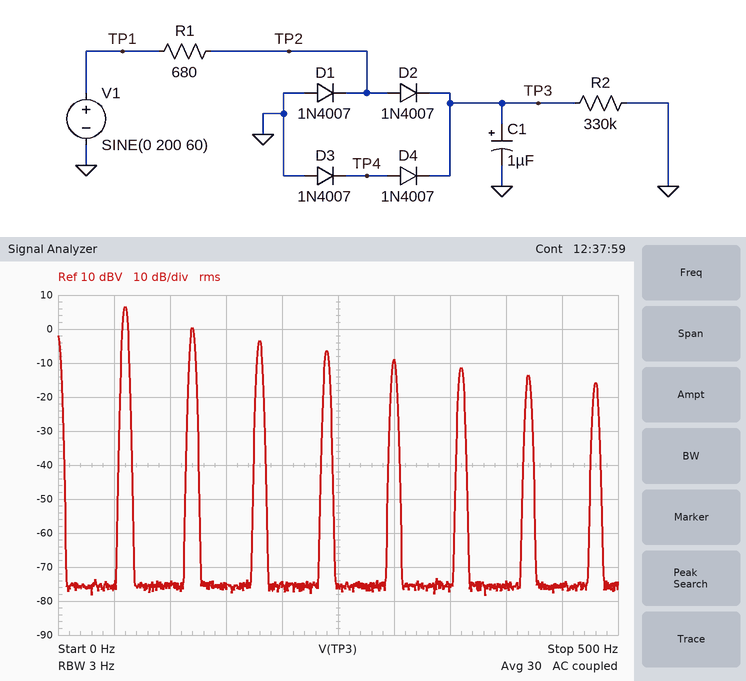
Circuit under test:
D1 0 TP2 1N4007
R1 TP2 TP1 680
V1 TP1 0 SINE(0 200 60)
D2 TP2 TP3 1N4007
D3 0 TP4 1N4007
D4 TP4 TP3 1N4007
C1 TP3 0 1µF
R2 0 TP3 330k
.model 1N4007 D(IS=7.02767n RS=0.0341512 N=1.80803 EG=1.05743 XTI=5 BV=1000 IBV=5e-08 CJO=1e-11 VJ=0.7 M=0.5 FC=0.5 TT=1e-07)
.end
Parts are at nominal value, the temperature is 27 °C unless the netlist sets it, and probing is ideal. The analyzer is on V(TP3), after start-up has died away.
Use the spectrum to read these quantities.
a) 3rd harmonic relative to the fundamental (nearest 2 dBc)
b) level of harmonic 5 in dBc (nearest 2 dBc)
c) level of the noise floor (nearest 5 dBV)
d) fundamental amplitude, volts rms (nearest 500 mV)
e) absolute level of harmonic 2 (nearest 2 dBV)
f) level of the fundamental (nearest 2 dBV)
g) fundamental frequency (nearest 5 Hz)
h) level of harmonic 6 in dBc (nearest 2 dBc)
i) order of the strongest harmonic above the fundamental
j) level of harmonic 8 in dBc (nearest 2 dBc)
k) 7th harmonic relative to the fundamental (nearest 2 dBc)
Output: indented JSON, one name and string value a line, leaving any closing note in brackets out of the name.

{
  "3rd harmonic relative to the fundamental": "-10 dBc",
  "level of harmonic 5 in dBc": "-16 dBc",
  "level of the noise floor": "-75 dBV",
  "fundamental amplitude, volts rms": "2.0 V",
  "absolute level of harmonic 2": "0 dBV",
  "level of the fundamental": "6 dBV",
  "fundamental frequency": "60 Hz",
  "level of harmonic 6 in dBc": "-18 dBc",
  "order of the strongest harmonic above the fundamental": "2",
  "level of harmonic 8 in dBc": "-22 dBc",
  "7th harmonic relative to the fundamental": "-20 dBc"
}
